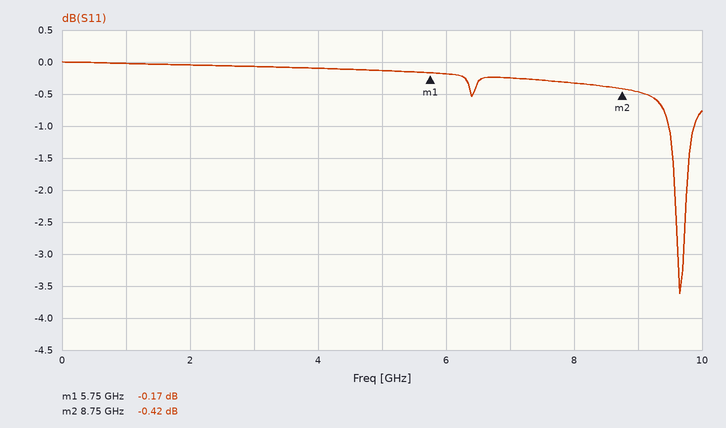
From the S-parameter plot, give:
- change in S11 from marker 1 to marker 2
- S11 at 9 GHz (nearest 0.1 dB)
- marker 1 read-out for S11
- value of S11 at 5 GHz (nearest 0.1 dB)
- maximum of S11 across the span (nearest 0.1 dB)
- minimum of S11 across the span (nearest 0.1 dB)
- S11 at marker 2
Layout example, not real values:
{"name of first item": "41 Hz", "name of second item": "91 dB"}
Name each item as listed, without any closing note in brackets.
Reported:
{"change in S11 from marker 1 to marker 2": "-0.25 dB", "S11 at 9 GHz": "-0.5 dB", "marker 1 read-out for S11": "-0.17 dB", "value of S11 at 5 GHz": "-0.1 dB", "maximum of S11 across the span": "0.0 dB", "minimum of S11 across the span": "-3.6 dB", "S11 at marker 2": "-0.42 dB"}
